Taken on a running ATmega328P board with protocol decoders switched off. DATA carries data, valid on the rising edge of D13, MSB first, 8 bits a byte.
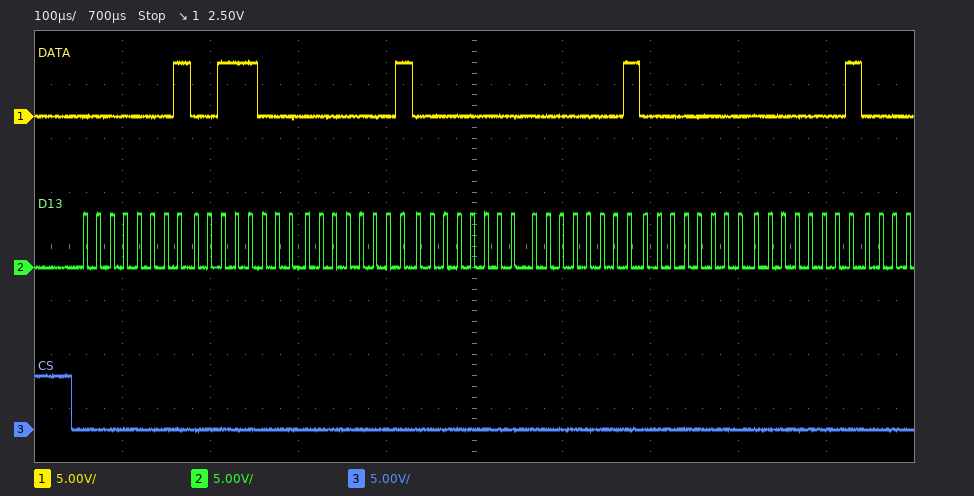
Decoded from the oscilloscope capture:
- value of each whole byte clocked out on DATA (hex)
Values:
01 38 01 00 01 00 01
